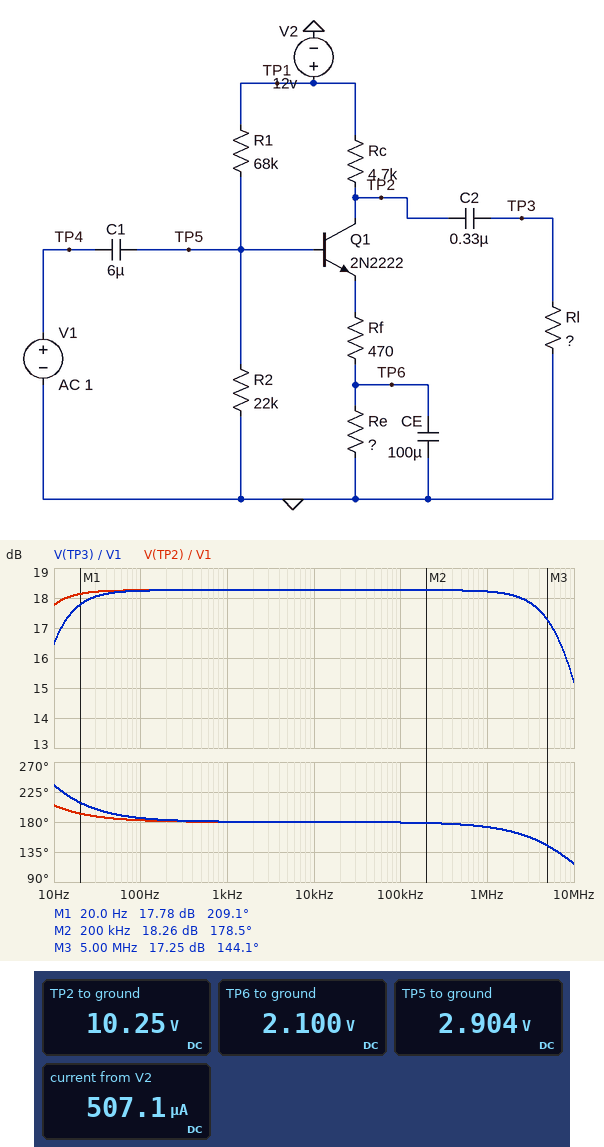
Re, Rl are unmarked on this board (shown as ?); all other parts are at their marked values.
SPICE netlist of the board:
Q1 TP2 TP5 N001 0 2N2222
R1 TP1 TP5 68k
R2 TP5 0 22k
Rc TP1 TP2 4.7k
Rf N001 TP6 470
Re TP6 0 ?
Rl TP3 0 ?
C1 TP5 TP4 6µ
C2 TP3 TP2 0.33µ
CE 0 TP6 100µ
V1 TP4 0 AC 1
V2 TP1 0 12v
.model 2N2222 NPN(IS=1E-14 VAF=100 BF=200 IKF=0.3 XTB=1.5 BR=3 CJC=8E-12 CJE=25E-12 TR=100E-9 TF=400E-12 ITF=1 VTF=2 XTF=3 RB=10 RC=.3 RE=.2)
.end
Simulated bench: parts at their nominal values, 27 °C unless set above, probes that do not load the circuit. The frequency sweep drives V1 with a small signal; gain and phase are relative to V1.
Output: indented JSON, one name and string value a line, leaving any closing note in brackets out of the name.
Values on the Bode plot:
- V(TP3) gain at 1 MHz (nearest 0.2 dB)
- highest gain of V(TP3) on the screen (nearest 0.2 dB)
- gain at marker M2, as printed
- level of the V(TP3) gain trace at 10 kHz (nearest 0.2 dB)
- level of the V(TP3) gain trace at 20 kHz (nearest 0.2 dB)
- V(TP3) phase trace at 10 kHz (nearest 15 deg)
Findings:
{
  "V(TP3) gain at 1 MHz": "18.2 dB",
  "highest gain of V(TP3) on the screen": "18.2 dB",
  "gain at marker M2, as printed": "18.26 dB",
  "level of the V(TP3) gain trace at 10 kHz": "18.2 dB",
  "level of the V(TP3) gain trace at 20 kHz": "18.2 dB",
  "V(TP3) phase trace at 10 kHz": "180 deg"
}
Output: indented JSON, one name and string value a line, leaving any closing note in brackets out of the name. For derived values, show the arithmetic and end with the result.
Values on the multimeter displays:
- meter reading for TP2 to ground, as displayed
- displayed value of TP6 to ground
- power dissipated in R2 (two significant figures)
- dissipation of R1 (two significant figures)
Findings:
{
  "meter reading for TP2 to ground, as displayed": "10.25 V",
  "displayed value of TP6 to ground": "2.100 V",
  "power dissipated in R2": "(2.904 V)^2 / 22 kΩ = 380 µW",
  "dissipation of R1": "(12 V - 2.904 V)^2 / 68 kΩ = 1.2 mW"
}
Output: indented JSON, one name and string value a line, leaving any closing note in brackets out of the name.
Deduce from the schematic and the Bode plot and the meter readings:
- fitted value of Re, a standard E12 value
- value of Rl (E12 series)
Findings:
{
  "fitted value of Re, a standard E12 value": "5.6 kΩ",
  "value of Rl": "82 kΩ"
}
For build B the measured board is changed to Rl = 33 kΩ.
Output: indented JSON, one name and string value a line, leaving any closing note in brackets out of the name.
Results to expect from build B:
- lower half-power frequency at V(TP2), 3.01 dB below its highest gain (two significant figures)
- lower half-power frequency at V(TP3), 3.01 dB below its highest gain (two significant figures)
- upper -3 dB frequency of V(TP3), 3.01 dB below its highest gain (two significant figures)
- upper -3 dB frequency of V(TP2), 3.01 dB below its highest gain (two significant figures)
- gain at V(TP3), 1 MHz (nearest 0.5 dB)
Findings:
{
  "lower half-power frequency at V(TP2), 3.01 dB below its highest gain": "3.5 Hz",
  "lower half-power frequency at V(TP3), 3.01 dB below its highest gain": "14 Hz",
  "upper -3 dB frequency of V(TP3), 3.01 dB below its highest gain": "11 MHz",
  "upper -3 dB frequency of V(TP2), 3.01 dB below its highest gain": "10 MHz",
  "gain at V(TP3), 1 MHz": "17.5 dB"
}
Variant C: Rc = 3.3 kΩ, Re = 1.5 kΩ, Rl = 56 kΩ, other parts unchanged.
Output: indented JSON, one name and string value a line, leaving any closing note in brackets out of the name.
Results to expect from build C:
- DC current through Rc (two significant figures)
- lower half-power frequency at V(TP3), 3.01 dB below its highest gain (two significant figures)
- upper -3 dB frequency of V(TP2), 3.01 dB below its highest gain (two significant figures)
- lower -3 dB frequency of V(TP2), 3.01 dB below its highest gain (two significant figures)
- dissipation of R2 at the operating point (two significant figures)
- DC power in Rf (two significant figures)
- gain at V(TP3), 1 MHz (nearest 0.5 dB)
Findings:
{
  "DC current through Rc": "1.1 mA",
  "lower half-power frequency at V(TP3), 3.01 dB below its highest gain": "10 Hz",
  "upper -3 dB frequency of V(TP2), 3.01 dB below its highest gain": "13 MHz",
  "lower -3 dB frequency of V(TP2), 3.01 dB below its highest gain": "4.5 Hz",
  "dissipation of R2 at the operating point": "370 µW",
  "DC power in Rf": "580 µW",
  "gain at V(TP3), 1 MHz": "16.0 dB"
}
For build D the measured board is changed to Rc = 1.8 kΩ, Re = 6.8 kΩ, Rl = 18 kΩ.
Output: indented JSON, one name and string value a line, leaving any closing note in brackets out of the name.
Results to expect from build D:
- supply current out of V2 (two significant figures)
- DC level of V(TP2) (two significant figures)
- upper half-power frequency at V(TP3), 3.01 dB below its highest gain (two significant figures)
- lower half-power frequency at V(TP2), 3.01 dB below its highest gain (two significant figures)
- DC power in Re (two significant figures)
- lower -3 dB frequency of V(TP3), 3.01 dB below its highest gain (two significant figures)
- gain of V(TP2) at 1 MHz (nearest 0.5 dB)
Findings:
{
  "supply current out of V2": "450 µA",
  "DC level of V(TP2)": "11 V",
  "upper half-power frequency at V(TP3), 3.01 dB below its highest gain": "33 MHz",
  "lower half-power frequency at V(TP2), 3.01 dB below its highest gain": "3.6 Hz",
  "DC power in Re": "670 µW",
  "lower -3 dB frequency of V(TP3), 3.01 dB below its highest gain": "25 Hz",
  "gain of V(TP2) at 1 MHz": "9.5 dB"
}
